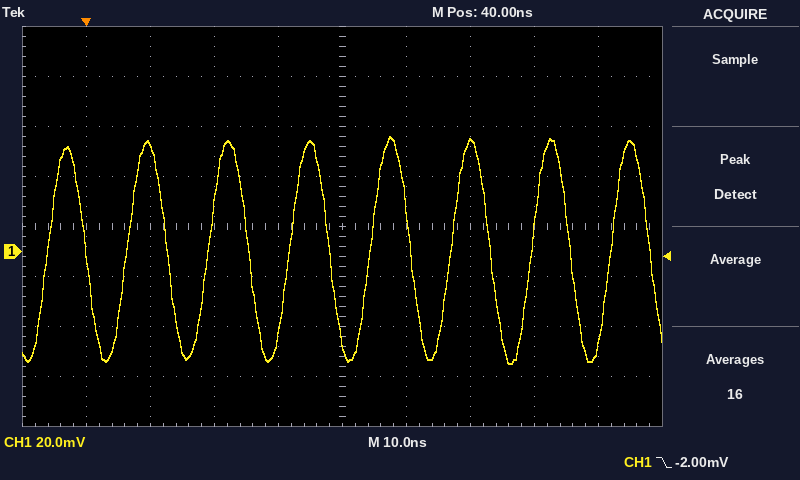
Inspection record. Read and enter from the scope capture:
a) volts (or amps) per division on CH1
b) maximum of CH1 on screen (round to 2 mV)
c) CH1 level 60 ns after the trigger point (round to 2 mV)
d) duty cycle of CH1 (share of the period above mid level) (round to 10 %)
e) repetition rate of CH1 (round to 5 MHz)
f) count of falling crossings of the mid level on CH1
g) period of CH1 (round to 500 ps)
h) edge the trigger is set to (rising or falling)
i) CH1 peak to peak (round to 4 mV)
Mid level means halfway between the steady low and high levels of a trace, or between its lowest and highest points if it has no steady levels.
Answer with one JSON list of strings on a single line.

["20 mV", "46 mV", "44 mV", "50 %", "80 MHz", "8", "12.5 ns", "falling", "92 mV"]
